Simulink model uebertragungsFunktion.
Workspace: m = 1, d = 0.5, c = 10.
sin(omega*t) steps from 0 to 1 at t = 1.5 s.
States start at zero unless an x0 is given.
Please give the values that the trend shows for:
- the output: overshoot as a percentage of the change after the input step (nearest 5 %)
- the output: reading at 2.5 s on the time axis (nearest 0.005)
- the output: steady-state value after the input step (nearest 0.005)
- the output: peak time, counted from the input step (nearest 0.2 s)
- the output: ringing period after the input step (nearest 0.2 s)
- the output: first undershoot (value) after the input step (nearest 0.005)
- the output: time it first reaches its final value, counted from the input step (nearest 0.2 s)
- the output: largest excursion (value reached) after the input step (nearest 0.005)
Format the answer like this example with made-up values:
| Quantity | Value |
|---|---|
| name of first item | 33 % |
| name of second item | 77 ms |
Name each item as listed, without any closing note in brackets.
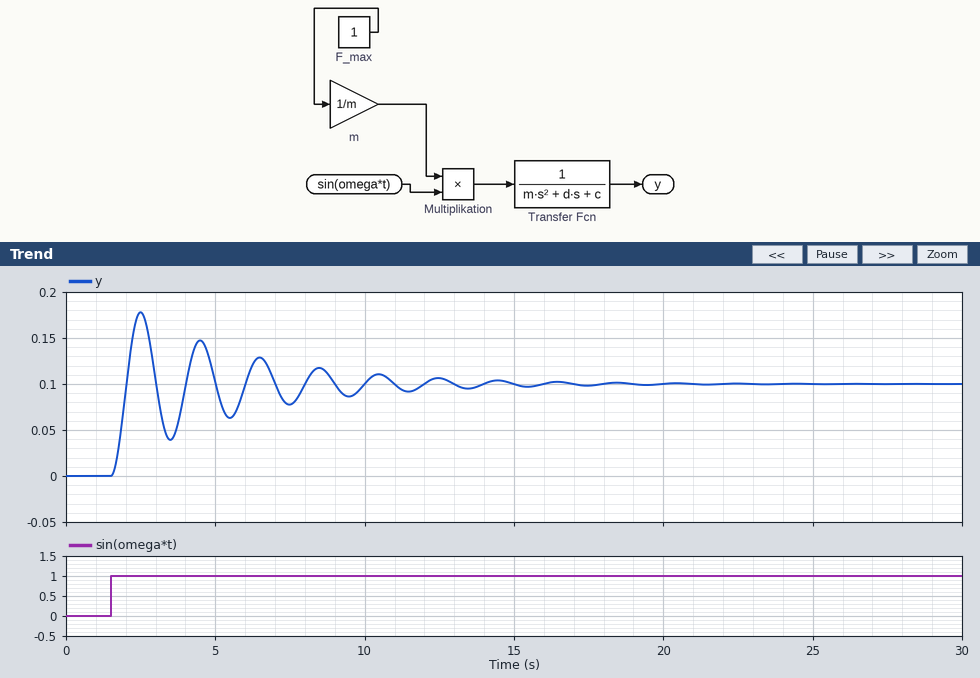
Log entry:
| Quantity | Value |
|---|---|
| the output: overshoot as a percentage of the change after the input step | 80 % |
| the output: reading at 2.5 s on the time axis | 0.180 |
| the output: steady-state value after the input step | 0.100 |
| the output: peak time, counted from the input step | 1.0 s |
| the output: ringing period after the input step | 2.0 s |
| the output: first undershoot (value) after the input step | 0.040 |
| the output: time it first reaches its final value, counted from the input step | 0.6 s |
| the output: largest excursion (value reached) after the input step | 0.180 |
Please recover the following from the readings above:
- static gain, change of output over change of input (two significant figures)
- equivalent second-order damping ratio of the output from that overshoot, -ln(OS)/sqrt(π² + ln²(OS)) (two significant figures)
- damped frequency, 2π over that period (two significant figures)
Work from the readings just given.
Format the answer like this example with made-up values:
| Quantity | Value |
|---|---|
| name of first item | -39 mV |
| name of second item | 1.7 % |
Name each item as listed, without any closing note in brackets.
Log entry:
| Quantity | Value |
|---|---|
| static gain, change of output over change of input | 0.10 |
| equivalent second-order damping ratio of the output from that overshoot, -ln(OS)/sqrt(π² + ln²(OS)) | 0.071 |
| damped frequency, 2π over that period | 3.1 rad/s |
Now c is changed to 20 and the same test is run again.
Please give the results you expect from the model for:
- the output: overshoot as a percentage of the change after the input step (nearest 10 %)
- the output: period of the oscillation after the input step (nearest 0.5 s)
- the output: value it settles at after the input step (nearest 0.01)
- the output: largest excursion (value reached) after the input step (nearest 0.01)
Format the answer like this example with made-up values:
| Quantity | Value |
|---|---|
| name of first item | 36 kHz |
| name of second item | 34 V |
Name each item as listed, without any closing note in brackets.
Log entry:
| Quantity | Value |
|---|---|
| the output: overshoot as a percentage of the change after the input step | 80 % |
| the output: period of the oscillation after the input step | 1.5 s |
| the output: value it settles at after the input step | 0.05 |
| the output: largest excursion (value reached) after the input step | 0.09 |
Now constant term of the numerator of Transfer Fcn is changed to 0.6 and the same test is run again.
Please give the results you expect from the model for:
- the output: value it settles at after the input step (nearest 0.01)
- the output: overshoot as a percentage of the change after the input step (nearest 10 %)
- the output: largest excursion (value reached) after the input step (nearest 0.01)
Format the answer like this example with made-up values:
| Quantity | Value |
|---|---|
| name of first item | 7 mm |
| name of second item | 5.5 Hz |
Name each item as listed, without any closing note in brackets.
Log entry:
| Quantity | Value |
|---|---|
| the output: value it settles at after the input step | 0.06 |
| the output: overshoot as a percentage of the change after the input step | 80 % |
| the output: largest excursion (value reached) after the input step | 0.11 |
